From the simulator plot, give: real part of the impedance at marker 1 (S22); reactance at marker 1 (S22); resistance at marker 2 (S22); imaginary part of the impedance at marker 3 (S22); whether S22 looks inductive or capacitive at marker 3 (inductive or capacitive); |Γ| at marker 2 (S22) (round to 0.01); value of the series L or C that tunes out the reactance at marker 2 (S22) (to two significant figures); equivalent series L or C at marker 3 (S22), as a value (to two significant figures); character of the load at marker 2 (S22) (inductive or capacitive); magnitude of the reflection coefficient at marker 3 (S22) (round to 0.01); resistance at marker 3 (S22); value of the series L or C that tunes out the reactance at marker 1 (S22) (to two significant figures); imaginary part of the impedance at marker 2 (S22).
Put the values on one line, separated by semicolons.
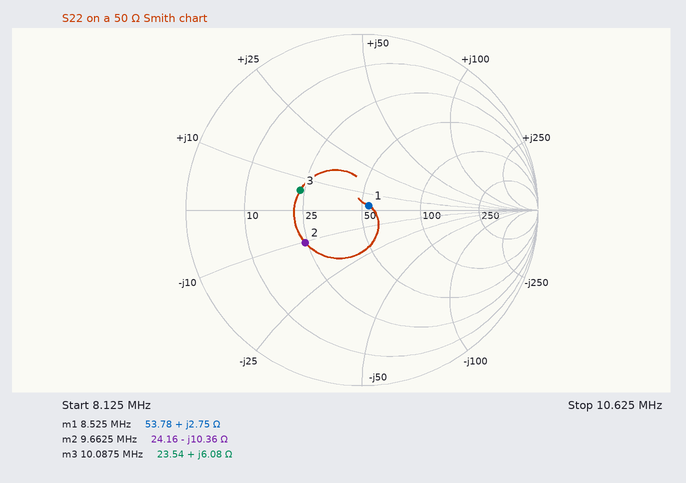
53.78 Ω; +2.75 Ω; 24.16 Ω; +6.08 Ω; inductive; 0.37; 170 nH; 96 nH; capacitive; 0.37; 23.54 Ω; 6.8 nF; -10.36 Ω
